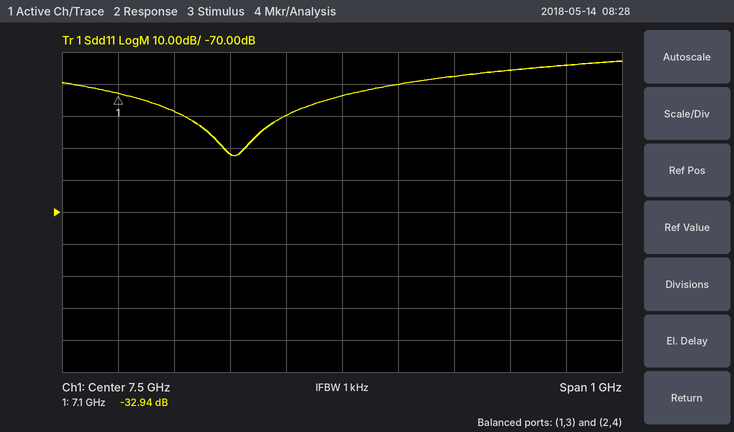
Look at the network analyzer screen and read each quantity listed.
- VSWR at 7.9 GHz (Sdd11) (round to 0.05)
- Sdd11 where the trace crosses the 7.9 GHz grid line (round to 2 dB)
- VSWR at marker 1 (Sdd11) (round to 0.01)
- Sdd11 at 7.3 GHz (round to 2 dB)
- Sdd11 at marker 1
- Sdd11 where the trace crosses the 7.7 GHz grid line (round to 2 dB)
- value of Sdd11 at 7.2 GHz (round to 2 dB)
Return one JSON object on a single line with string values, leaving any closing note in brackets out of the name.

{"VSWR at 7.9 GHz (Sdd11)": "1.15", "Sdd11 where the trace crosses the 7.9 GHz grid line": "-24 dB", "VSWR at marker 1 (Sdd11)": "1.05", "Sdd11 at 7.3 GHz": "-52 dB", "Sdd11 at marker 1": "-32.94 dB", "Sdd11 where the trace crosses the 7.7 GHz grid line": "-28 dB", "value of Sdd11 at 7.2 GHz": "-38 dB"}
